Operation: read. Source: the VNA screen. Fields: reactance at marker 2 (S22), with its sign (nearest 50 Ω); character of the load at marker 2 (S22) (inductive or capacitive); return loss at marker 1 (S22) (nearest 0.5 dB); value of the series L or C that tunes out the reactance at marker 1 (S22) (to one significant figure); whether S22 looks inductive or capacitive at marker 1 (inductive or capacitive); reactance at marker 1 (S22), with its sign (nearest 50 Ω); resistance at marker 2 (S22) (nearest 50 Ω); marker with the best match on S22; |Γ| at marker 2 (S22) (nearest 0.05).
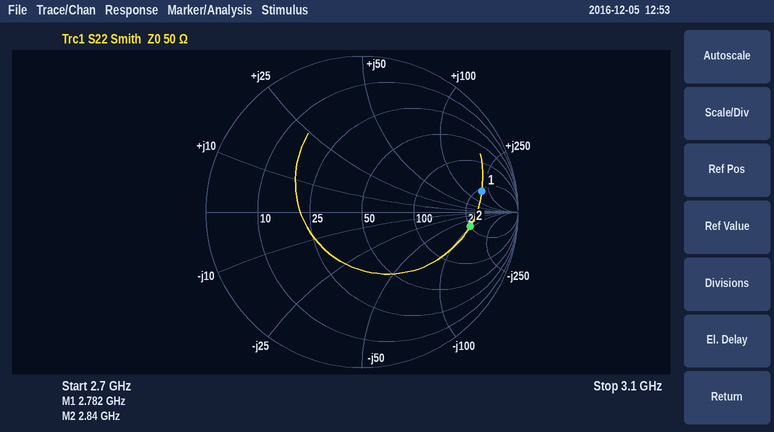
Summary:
-100 Ω
capacitive
2.0 dB
300 fF
inductive
+200 Ω
250 Ω
marker 2
0.70
